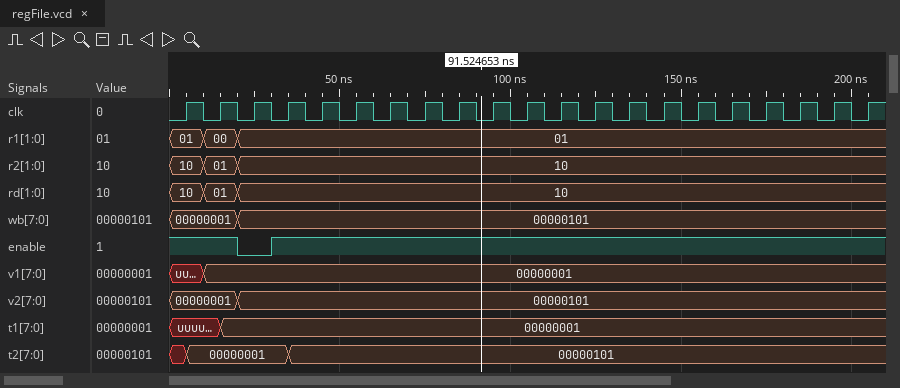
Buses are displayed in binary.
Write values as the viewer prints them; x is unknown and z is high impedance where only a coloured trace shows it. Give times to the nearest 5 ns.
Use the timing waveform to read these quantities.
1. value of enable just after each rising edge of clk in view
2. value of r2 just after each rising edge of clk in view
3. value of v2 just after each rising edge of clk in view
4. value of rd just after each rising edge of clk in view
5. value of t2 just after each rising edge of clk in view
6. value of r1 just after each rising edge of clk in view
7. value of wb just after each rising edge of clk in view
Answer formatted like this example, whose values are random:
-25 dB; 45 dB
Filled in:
1 1 0 1 1 1 1 1 1 1 1 1 1 1 1 1 1 1 1 1 1; 10, 01, 10, 10, 10, 10, 10, 10, 10, 10, 10, 10, 10, 10, 10, 10, 10, 10, 10, 10, 10; 00000001, 00000001, 00000101, 00000101, 00000101, 00000101, 00000101, 00000101, 00000101, 00000101, 00000101, 00000101, 00000101, 00000101, 00000101, 00000101, 00000101, 00000101, 00000101, 00000101, 00000101; 10, 01, 10, 10, 10, 10, 10, 10, 10, 10, 10, 10, 10, 10, 10, 10, 10, 10, 10, 10, 10; 00000001, 00000001, 00000001, 00000101, 00000101, 00000101, 00000101, 00000101, 00000101, 00000101, 00000101, 00000101, 00000101, 00000101, 00000101, 00000101, 00000101, 00000101, 00000101, 00000101, 00000101; 01, 00, 01, 01, 01, 01, 01, 01, 01, 01, 01, 01, 01, 01, 01, 01, 01, 01, 01, 01, 01; 00000001, 00000001, 00000101, 00000101, 00000101, 00000101, 00000101, 00000101, 00000101, 00000101, 00000101, 00000101, 00000101, 00000101, 00000101, 00000101, 00000101, 00000101, 00000101, 00000101, 00000101
